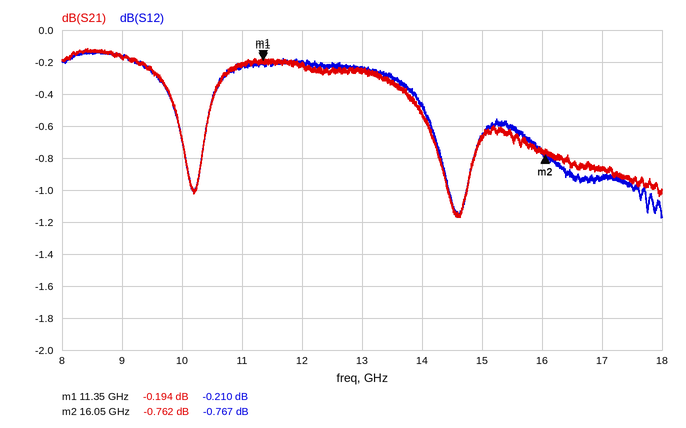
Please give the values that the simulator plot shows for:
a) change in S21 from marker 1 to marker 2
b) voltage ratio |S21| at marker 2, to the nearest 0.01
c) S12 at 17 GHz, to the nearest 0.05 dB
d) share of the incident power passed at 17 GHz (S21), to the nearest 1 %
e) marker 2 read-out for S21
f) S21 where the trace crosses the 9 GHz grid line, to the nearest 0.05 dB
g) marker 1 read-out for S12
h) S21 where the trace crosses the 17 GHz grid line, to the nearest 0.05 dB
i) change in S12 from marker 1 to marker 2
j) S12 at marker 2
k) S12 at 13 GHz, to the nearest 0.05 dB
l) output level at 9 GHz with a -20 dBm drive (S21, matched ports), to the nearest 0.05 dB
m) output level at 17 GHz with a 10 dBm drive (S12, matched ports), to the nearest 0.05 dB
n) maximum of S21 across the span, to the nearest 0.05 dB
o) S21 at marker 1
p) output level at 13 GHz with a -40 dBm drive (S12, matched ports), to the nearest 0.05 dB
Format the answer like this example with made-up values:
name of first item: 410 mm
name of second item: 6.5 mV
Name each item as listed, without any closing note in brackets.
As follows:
change in S21 from marker 1 to marker 2: -0.568 dB
voltage ratio |S21| at marker 2, to the nearest 0.01: 0.92
S12 at 17 GHz, to the nearest 0.05 dB: -0.90 dB
share of the incident power passed at 17 GHz (S21), to the nearest 1 %: 82 %
marker 2 read-out for S21: -0.762 dB
S21 where the trace crosses the 9 GHz grid line, to the nearest 0.05 dB: -0.15 dB
marker 1 read-out for S12: -0.210 dB
S21 where the trace crosses the 17 GHz grid line, to the nearest 0.05 dB: -0.85 dB
change in S12 from marker 1 to marker 2: -0.557 dB
S12 at marker 2: -0.767 dB
S12 at 13 GHz, to the nearest 0.05 dB: -0.25 dB
output level at 9 GHz with a -20 dBm drive (S21, matched ports), to the nearest 0.05 dB: -20.15 dBm
output level at 17 GHz with a 10 dBm drive (S12, matched ports), to the nearest 0.05 dB: 9.10 dBm
maximum of S21 across the span, to the nearest 0.05 dB: -0.10 dB
S21 at marker 1: -0.194 dB
output level at 13 GHz with a -40 dBm drive (S12, matched ports), to the nearest 0.05 dB: -40.25 dBm
